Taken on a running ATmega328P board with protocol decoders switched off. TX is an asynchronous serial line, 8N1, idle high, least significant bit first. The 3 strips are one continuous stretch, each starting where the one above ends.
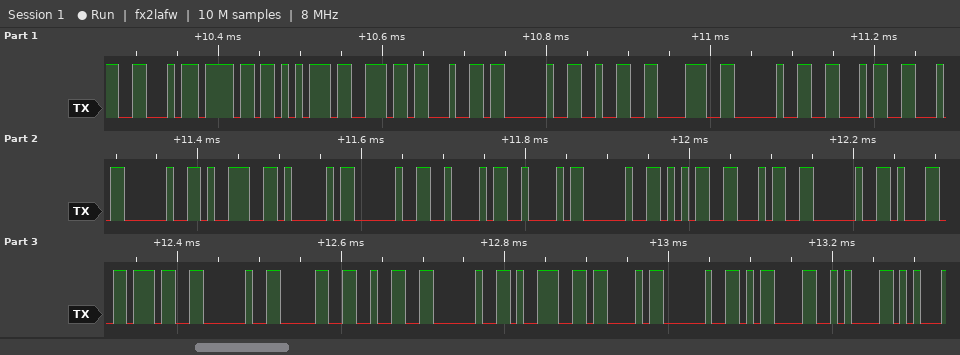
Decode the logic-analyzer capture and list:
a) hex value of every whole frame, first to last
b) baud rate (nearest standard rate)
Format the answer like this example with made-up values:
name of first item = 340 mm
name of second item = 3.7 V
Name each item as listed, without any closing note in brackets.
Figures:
hex value of every whole frame, first to last = 46 6F 75 6E 64 20 32 38 20 46 46 20 39 41 20 42 42 20 35 34 20 31 37 20 30 32 20 39 43 20 0D 0A
baud rate = 115200 baud
